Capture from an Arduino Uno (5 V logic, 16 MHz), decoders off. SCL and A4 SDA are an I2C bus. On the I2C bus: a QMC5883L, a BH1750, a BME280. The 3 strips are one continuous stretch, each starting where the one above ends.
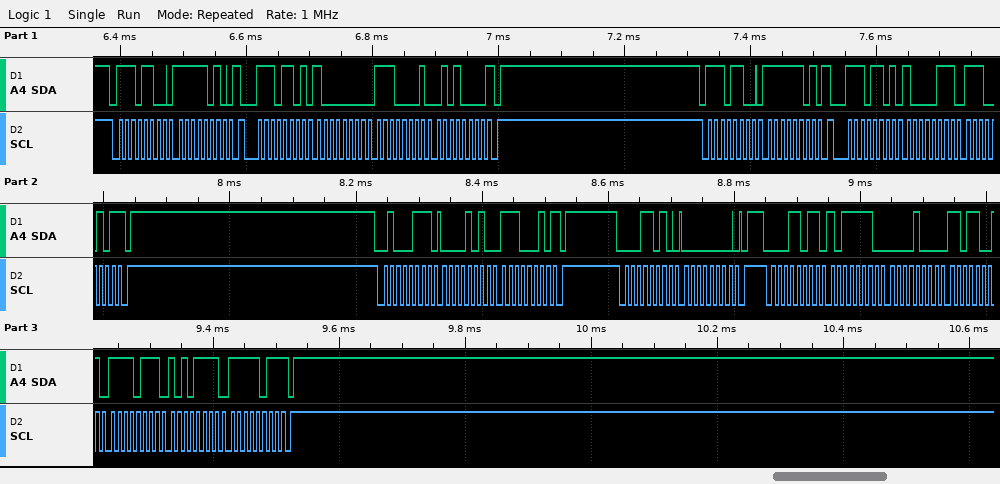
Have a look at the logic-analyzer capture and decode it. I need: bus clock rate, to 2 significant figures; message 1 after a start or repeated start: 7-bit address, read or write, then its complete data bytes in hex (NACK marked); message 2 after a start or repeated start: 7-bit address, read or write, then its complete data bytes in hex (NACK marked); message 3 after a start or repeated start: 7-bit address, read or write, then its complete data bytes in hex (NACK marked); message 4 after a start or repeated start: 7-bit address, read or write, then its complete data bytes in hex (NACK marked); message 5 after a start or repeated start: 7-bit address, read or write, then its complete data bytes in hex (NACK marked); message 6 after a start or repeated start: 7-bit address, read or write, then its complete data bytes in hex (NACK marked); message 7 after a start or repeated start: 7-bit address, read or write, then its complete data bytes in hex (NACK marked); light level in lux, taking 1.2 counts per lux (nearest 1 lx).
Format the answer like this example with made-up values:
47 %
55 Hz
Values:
100 kHz
0x76 write: FA
0x76 read: 80 E1 50 NACK
0x76 write: FD
0x76 read: 87 E5 NACK
0x23 read: 0A E2 NACK
0x0D write: 00
0x0D read: BE 08 D9 F7 AF FB NACK
2322 lx
